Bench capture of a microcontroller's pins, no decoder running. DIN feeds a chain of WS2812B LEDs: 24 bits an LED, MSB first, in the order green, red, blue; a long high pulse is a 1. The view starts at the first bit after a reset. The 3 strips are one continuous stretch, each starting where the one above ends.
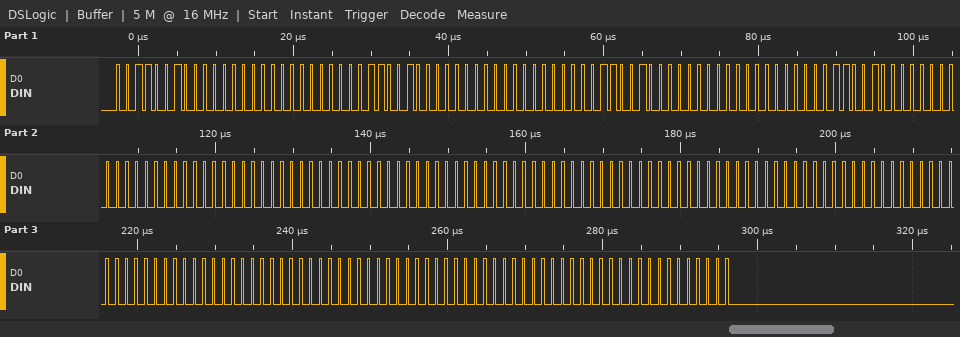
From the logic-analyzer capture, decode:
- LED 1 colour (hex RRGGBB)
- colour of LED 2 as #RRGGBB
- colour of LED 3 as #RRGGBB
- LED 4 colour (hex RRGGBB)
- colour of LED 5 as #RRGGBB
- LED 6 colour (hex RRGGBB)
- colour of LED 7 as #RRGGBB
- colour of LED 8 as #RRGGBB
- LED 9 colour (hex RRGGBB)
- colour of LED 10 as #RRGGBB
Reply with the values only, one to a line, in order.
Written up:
#003200
#003200
#003200
#003200
#000000
#000000
#000000
#000000
#000000
#000000
